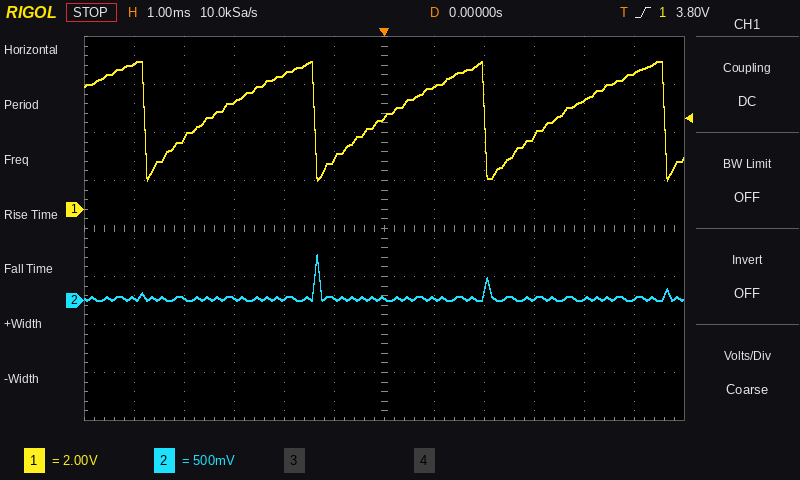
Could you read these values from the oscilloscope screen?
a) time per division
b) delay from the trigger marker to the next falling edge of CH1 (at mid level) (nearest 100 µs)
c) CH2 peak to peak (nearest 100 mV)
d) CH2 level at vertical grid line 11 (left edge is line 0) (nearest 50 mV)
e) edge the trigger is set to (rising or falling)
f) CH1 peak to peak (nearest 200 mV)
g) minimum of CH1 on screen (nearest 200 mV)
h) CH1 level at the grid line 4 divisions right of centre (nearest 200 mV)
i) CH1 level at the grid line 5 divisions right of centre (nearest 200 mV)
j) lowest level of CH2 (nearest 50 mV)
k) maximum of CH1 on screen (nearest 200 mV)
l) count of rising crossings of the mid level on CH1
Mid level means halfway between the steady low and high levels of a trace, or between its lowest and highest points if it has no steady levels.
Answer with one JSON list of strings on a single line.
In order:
["1 ms", "2.0 ms", "500 mV", "0 mV", "rising", "5.0 V", "1.2 V", "4.6 V", "5.6 V", "0 mV", "6.2 V", "3"]
